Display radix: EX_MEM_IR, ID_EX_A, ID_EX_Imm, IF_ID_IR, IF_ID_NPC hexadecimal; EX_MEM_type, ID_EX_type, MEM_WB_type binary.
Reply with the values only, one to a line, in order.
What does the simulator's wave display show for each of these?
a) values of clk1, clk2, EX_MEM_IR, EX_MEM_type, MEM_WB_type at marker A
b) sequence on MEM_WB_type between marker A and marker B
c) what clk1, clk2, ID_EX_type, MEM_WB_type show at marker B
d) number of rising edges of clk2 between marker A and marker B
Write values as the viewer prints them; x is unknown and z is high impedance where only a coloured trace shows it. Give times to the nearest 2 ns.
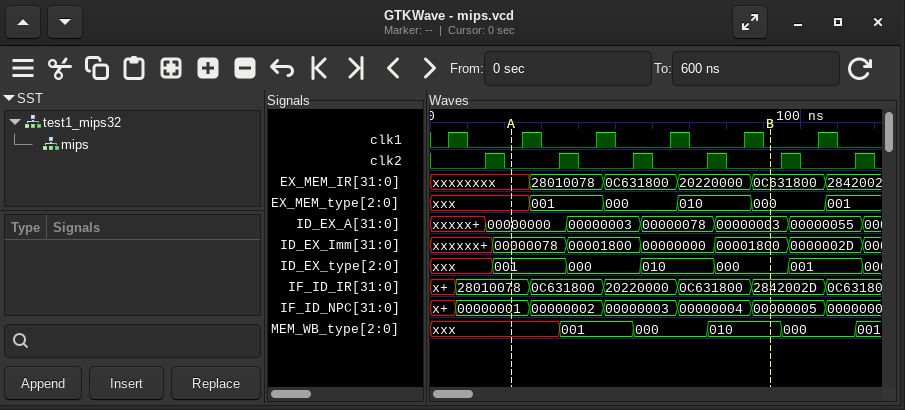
clk1=0, clk2=0, EX_MEM_IR=xxxxxxxx, EX_MEM_type=xxx, MEM_WB_type=xxx
xxx, 001, 000, 010
clk1=0, clk2=0, ID_EX_type=000, MEM_WB_type=010
3
